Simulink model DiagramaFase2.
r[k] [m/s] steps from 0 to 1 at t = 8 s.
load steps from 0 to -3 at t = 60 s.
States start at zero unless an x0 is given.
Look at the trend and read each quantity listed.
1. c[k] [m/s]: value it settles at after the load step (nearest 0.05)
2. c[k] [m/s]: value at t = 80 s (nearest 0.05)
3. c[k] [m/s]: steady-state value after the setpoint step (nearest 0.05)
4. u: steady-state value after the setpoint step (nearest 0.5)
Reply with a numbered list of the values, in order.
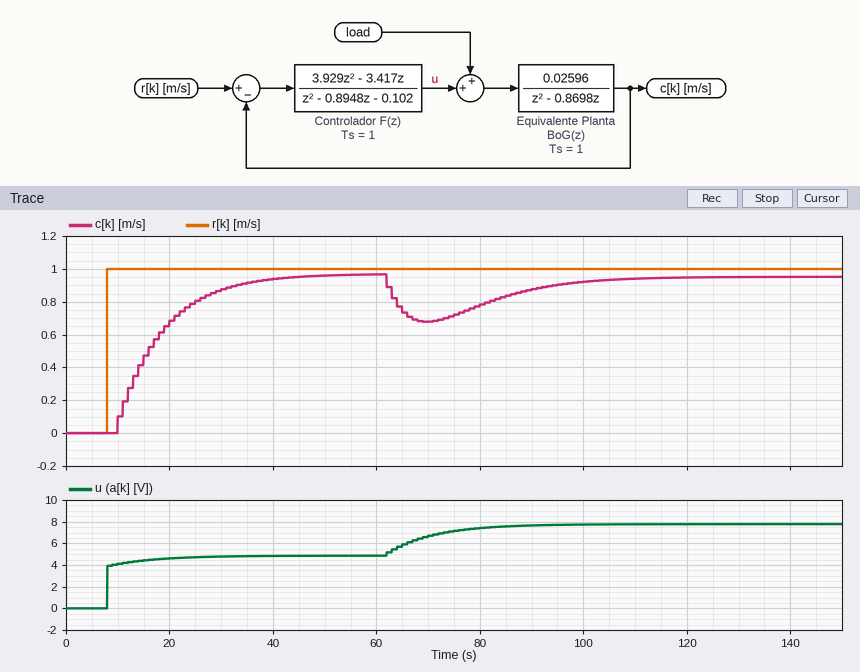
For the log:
1. 0.95
2. 0.80
3. 0.95
4. 5.0
